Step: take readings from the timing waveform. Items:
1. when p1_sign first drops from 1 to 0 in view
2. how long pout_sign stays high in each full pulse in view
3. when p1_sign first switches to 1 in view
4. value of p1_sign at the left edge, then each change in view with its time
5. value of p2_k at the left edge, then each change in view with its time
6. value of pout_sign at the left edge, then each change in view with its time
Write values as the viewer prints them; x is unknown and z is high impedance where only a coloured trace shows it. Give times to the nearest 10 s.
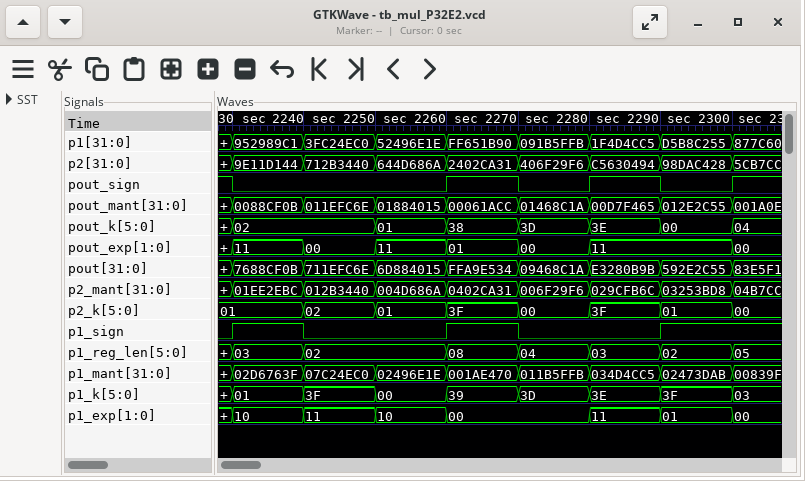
2240 s
10 s, 10 s
2230 s
0, 1 at 2230 s, 0 at 2240 s, 1 at 2260 s, 0 at 2270 s, 1 at 2290 s
01, 02 at 2240 s, 01 at 2250 s, 3F at 2260 s, 00 at 2270 s, 3F at 2280 s, 01 at 2290 s, 00 at 2300 s
1, 0 at 2230 s, 1 at 2260 s, 0 at 2270 s, 1 at 2280 s, 0 at 2290 s, 1 at 2300 s
